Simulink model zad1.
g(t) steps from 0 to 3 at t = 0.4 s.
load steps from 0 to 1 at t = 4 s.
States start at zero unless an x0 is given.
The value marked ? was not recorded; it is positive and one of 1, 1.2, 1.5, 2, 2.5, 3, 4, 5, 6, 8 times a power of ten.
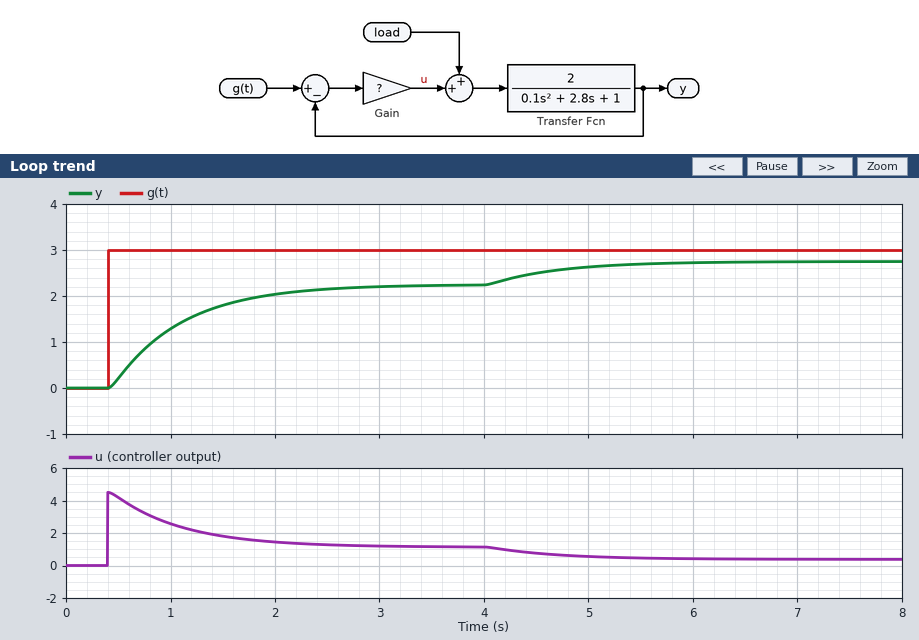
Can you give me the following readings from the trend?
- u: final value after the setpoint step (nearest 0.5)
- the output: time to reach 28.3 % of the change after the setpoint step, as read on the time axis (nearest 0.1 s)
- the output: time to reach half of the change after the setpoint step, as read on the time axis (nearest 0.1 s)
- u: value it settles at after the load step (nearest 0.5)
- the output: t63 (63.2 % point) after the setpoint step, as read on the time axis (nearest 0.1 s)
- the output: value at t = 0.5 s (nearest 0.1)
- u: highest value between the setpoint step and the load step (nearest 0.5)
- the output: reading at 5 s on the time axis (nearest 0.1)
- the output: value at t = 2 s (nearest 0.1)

1.0
0.7 s
0.9 s
0.5
1.1 s
0.2
4.5
2.6
2.0
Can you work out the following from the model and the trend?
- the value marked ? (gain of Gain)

1.5
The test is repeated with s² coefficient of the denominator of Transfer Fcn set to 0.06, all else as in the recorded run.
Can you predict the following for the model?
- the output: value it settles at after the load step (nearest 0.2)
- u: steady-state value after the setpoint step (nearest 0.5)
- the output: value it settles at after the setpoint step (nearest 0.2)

2.8
1.0
2.2
